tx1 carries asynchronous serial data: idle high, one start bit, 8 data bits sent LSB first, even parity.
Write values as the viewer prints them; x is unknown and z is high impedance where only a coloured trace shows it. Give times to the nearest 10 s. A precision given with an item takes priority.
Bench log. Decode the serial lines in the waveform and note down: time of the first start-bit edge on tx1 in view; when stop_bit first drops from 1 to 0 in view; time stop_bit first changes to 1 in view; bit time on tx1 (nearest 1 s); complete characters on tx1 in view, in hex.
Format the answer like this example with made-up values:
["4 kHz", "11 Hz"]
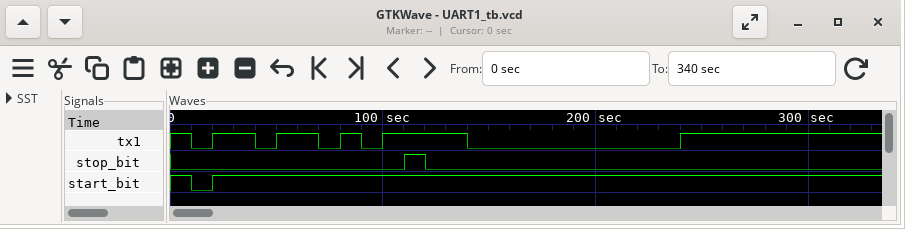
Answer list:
["10 s", "120 s", "110 s", "10 s", "5B, 00"]
